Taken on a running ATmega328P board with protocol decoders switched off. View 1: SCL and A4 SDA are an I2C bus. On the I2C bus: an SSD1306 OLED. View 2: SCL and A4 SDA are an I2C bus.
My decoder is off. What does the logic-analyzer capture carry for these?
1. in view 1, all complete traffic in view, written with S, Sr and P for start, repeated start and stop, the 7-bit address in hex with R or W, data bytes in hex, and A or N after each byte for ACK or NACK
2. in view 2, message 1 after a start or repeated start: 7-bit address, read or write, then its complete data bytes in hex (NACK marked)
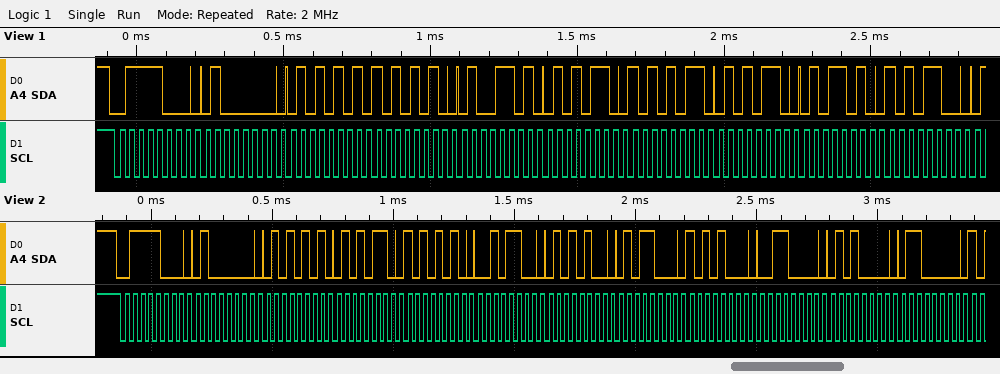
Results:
S 3CW A 40 A 55 A AA A 4D A 56 A AB A 56 A 5A A AC A
0x3C write: 40 55 56 AA 2C 54 58 A8 30 50 60
